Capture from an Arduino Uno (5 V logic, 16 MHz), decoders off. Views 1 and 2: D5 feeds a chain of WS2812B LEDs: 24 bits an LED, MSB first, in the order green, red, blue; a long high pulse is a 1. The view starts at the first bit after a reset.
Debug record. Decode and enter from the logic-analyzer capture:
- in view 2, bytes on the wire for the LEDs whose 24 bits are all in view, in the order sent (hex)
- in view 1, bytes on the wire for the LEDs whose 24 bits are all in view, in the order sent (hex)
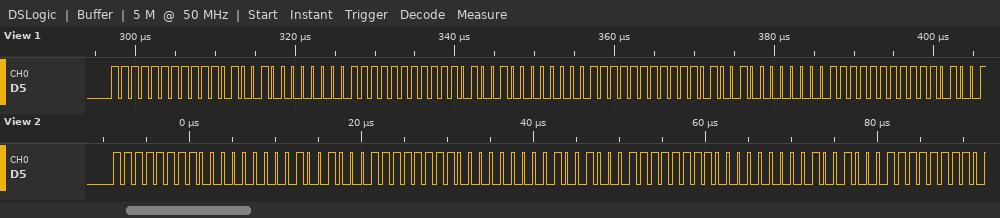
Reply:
FF 00 48 FF 00 48 FF 00 48
FF E9 00 FF E9 00 FF E9 00
